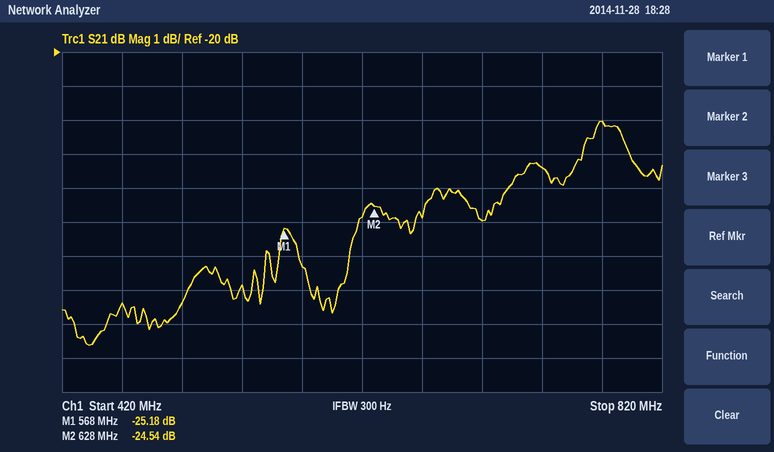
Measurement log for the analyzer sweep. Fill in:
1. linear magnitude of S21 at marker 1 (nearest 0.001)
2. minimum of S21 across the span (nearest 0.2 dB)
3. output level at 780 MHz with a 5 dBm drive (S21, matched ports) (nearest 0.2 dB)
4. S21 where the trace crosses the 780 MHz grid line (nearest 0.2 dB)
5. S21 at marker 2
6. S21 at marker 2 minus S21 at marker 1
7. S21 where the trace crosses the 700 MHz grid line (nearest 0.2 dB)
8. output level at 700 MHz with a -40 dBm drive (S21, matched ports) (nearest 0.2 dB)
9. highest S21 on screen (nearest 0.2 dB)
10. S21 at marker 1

0.055
-28.6 dB
-17.0 dBm
-22.0 dB
-24.54 dB
0.64 dB
-25.0 dB
-65.0 dBm
-22.0 dB
-25.18 dB
